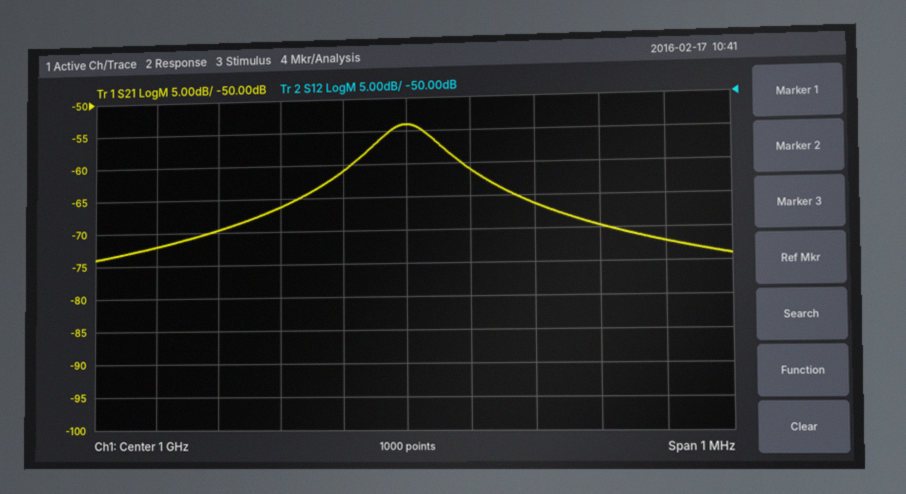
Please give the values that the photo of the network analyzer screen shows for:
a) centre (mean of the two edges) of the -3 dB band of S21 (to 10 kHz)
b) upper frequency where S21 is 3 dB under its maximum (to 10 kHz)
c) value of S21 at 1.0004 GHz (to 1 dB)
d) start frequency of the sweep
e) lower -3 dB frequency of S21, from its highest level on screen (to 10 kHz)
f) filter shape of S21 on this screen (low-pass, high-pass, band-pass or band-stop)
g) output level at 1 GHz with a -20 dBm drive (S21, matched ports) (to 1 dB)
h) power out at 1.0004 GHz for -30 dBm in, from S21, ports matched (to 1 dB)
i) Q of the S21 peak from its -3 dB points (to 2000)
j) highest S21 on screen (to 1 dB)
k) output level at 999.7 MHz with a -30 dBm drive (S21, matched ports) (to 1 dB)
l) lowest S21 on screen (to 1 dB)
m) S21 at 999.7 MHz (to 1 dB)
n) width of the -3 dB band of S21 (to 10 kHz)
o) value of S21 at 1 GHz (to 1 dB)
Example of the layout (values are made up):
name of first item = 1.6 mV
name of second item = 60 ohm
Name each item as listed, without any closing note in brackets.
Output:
centre (mean of the two edges) of the -3 dB band of S21 = 1.00000 GHz
upper frequency where S21 is 3 dB under its maximum = 1.00005 GHz
value of S21 at 1.0004 GHz = -72 dB
start frequency of the sweep = 999.5 MHz
lower -3 dB frequency of S21, from its highest level on screen = 999.95 MHz
filter shape of S21 on this screen = band-pass
output level at 1 GHz with a -20 dBm drive (S21, matched ports) = -74 dBm
power out at 1.0004 GHz for -30 dBm in, from S21, ports matched = -102 dBm
Q of the S21 peak from its -3 dB points = 10000
highest S21 on screen = -54 dB
output level at 999.7 MHz with a -30 dBm drive (S21, matched ports) = -100 dBm
lowest S21 on screen = -74 dB
S21 at 999.7 MHz = -70 dB
width of the -3 dB band of S21 = 100 kHz
value of S21 at 1 GHz = -54 dB
